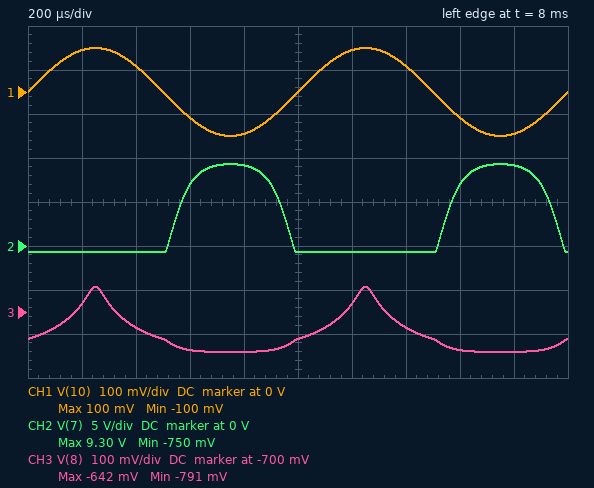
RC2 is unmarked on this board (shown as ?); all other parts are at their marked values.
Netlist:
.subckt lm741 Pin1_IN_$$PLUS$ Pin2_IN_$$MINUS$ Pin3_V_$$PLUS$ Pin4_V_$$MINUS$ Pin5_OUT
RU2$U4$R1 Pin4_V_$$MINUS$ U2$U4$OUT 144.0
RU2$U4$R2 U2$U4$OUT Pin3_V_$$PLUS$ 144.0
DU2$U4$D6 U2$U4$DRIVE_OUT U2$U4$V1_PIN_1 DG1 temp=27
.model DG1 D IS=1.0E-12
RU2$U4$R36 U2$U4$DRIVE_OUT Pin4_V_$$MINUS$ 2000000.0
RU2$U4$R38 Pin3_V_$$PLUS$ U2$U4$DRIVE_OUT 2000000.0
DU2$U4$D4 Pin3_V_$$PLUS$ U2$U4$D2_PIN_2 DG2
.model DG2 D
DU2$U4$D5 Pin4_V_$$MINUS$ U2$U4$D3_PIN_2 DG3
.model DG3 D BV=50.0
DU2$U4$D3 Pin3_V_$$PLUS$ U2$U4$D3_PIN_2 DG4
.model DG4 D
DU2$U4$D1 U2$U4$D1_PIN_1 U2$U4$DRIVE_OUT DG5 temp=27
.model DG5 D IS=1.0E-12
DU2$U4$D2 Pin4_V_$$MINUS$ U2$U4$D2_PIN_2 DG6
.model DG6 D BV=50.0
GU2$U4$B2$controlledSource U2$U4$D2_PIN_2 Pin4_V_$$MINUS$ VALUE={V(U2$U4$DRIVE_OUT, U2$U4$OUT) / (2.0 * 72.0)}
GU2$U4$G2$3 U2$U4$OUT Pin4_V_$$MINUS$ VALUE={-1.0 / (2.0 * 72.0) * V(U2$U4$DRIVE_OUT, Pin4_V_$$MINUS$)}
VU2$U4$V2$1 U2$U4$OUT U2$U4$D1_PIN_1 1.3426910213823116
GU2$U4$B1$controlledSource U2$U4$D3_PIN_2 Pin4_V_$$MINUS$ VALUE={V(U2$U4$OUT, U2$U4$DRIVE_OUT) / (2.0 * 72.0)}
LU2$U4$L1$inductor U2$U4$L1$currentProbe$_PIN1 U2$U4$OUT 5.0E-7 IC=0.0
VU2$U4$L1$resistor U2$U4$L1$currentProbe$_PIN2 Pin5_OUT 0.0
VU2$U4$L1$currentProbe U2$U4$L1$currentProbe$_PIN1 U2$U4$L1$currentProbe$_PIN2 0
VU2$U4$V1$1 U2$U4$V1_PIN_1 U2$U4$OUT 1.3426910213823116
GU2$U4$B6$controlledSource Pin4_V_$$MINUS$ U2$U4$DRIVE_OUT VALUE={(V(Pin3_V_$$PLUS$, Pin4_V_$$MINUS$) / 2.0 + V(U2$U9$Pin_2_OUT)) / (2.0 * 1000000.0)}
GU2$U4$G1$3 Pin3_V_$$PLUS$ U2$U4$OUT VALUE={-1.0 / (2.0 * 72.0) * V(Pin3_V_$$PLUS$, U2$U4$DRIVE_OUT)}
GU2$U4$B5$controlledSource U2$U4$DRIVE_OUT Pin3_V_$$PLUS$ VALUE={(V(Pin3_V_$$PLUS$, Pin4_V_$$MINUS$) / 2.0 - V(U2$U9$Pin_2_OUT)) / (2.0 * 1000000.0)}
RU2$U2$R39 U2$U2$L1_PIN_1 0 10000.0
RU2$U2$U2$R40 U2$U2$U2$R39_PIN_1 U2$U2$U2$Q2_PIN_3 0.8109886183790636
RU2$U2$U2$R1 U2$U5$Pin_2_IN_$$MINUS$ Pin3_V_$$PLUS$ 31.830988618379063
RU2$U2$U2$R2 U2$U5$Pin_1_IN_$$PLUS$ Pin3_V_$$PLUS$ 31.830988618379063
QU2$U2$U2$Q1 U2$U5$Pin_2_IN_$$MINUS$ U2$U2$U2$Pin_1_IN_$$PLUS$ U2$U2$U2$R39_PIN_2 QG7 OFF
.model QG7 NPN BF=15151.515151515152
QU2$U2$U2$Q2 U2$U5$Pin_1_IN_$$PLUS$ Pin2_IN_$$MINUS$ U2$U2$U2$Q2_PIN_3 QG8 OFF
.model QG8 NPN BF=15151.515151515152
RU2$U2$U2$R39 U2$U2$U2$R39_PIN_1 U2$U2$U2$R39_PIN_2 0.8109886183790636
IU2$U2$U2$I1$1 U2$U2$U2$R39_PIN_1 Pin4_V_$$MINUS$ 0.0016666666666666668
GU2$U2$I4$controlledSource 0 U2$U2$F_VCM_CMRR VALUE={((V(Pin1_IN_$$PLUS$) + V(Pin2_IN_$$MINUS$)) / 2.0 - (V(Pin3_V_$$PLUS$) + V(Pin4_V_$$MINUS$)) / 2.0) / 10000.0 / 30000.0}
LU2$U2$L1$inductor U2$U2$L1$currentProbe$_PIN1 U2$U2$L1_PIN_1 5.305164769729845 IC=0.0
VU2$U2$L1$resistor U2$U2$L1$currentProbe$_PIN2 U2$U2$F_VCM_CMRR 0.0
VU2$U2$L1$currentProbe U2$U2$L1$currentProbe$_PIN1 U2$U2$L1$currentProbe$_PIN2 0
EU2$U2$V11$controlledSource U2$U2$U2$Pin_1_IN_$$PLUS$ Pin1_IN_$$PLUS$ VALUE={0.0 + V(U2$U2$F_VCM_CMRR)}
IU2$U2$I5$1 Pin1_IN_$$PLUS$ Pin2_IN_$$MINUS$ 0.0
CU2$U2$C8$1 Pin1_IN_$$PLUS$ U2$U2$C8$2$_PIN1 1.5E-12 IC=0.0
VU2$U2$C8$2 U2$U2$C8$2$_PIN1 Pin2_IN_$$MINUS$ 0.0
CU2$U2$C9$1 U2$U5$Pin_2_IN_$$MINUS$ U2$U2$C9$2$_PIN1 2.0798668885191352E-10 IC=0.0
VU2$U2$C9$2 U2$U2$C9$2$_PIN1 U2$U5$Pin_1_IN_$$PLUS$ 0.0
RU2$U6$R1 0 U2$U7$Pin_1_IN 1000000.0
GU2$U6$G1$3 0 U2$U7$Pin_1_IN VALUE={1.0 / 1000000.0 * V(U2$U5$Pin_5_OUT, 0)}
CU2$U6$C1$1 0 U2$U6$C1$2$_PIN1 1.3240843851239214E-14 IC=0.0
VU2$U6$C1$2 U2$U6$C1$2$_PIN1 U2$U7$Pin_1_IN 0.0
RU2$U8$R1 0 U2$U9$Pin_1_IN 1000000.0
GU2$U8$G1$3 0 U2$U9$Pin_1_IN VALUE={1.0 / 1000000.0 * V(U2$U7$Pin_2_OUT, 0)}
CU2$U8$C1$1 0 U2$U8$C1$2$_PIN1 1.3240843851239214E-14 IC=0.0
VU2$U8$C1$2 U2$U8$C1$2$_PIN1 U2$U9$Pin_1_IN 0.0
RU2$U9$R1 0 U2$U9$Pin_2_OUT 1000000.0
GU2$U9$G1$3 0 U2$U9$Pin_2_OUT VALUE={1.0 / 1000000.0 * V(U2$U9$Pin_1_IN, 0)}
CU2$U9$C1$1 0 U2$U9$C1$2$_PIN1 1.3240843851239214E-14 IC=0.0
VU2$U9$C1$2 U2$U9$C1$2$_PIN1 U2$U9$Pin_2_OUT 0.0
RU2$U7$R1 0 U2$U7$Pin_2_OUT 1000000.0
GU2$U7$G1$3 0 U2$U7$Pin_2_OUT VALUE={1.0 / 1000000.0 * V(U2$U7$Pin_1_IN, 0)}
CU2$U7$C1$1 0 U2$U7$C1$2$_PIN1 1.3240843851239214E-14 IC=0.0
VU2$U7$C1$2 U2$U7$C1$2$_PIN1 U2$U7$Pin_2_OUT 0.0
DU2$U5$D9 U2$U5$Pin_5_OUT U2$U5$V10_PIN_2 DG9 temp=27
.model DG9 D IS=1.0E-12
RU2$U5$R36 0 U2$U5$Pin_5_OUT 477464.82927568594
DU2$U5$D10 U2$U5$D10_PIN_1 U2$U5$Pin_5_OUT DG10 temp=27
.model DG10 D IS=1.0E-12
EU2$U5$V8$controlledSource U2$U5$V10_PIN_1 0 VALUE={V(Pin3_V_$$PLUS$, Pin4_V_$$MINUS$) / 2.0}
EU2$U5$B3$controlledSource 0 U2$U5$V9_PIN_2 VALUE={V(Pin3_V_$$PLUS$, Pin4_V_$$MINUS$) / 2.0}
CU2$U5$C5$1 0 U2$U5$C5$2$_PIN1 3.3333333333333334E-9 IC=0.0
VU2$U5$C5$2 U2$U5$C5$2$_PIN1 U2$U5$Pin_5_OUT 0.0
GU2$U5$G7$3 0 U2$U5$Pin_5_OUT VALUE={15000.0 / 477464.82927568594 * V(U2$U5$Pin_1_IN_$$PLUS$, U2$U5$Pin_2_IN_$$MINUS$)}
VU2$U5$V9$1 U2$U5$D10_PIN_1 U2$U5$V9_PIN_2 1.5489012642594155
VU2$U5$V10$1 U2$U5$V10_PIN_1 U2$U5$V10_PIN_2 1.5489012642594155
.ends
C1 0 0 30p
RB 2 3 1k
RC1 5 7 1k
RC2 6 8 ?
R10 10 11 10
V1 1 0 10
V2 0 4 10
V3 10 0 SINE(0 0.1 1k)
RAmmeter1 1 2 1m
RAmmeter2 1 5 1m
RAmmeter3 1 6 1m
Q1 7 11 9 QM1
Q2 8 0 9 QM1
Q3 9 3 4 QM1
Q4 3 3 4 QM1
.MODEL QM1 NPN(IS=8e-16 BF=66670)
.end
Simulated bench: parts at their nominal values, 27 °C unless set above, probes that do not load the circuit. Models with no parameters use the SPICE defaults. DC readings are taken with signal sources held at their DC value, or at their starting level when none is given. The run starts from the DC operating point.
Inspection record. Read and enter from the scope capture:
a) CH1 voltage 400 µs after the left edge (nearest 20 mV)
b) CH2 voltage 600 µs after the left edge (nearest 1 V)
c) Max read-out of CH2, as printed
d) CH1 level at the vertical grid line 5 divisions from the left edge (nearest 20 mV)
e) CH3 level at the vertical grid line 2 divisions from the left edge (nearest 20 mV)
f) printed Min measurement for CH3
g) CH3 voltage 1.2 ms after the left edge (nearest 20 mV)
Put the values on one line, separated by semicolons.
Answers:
60 mV; 7 V; 9.30 V; 0 V; -740 mV; -791 mV; -680 mV
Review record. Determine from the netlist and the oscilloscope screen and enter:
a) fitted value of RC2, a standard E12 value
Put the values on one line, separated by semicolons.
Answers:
3.3 kΩ
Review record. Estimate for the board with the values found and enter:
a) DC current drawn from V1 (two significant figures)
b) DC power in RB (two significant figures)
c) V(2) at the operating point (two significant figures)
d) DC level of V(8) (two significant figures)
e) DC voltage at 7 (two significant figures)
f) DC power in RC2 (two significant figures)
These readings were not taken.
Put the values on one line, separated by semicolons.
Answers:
33 mA; 370 mW; 10 V; -760 mV; -700 mV; 35 mW
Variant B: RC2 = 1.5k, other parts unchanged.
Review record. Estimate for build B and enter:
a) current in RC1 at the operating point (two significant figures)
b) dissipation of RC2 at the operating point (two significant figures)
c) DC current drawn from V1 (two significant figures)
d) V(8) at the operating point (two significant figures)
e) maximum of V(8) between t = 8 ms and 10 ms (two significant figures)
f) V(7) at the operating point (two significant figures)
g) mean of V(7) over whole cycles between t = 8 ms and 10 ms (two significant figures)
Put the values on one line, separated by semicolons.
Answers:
10 mA; 77 mW; 37 mA; -730 mV; 5.1 V; -420 mV; 3.1 V
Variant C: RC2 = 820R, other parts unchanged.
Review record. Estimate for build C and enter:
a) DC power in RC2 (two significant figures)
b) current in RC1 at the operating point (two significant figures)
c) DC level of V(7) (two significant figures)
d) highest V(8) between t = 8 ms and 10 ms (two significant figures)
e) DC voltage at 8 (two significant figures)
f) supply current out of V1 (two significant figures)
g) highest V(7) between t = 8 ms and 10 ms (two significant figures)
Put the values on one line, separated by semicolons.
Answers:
76 mW; 9.6 mA; 400 mV; 7.3 V; 2.1 V; 38 mA; 9.5 V
